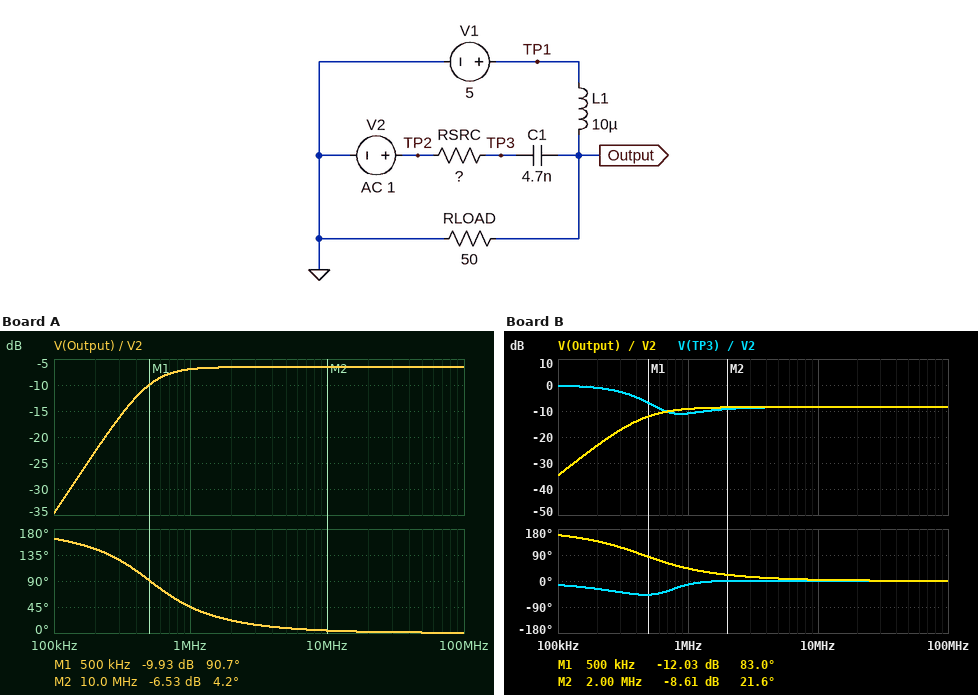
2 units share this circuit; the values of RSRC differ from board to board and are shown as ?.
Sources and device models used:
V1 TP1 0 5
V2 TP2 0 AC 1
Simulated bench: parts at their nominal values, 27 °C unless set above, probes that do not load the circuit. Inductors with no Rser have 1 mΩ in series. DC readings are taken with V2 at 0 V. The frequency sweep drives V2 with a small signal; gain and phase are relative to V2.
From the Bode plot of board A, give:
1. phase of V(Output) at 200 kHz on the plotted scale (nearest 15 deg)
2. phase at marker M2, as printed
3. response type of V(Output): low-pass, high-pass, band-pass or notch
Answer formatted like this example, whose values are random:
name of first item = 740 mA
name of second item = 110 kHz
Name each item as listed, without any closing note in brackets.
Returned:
phase of V(Output) at 200 kHz on the plotted scale = 150 deg
phase at marker M2, as printed = 4.2 deg
response type of V(Output): low-pass, high-pass, band-pass or notch = high-pass
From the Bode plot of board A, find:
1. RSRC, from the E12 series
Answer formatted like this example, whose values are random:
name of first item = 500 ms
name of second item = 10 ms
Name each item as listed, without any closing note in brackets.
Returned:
RSRC, from the E12 series = 56 Ω
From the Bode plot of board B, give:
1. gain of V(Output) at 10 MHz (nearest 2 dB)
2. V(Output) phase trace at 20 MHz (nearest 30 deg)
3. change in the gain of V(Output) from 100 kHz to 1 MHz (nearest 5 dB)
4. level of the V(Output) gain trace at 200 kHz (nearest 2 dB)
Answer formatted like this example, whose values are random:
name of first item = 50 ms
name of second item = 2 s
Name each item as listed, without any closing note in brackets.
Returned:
gain of V(Output) at 10 MHz = -8 dB
V(Output) phase trace at 20 MHz = 0 deg
change in the gain of V(Output) from 100 kHz to 1 MHz = 25 dB
level of the V(Output) gain trace at 200 kHz = -24 dB
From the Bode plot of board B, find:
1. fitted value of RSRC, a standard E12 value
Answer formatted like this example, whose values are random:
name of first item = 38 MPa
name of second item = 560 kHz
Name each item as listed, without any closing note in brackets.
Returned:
fitted value of RSRC, a standard E12 value = 82 Ω
